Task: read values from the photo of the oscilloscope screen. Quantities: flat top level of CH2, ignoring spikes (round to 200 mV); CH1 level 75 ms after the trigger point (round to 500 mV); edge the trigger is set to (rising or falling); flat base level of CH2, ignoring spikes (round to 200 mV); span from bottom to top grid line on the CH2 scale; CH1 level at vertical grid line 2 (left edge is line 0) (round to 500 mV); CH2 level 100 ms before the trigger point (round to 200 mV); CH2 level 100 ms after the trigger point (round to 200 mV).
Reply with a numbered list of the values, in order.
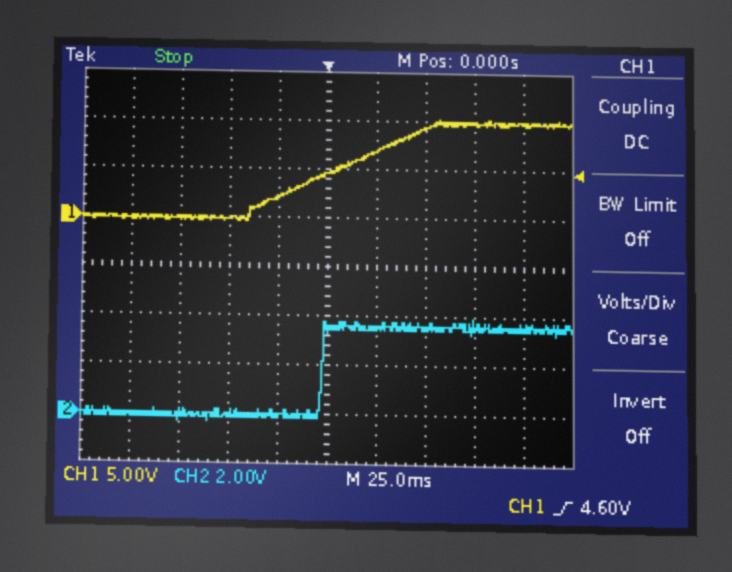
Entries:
1. 3.6 V
2. 10.0 V
3. rising
4. 0.0 V
5. 16 V
6. 0.0 V
7. 0.0 V
8. 3.6 V
